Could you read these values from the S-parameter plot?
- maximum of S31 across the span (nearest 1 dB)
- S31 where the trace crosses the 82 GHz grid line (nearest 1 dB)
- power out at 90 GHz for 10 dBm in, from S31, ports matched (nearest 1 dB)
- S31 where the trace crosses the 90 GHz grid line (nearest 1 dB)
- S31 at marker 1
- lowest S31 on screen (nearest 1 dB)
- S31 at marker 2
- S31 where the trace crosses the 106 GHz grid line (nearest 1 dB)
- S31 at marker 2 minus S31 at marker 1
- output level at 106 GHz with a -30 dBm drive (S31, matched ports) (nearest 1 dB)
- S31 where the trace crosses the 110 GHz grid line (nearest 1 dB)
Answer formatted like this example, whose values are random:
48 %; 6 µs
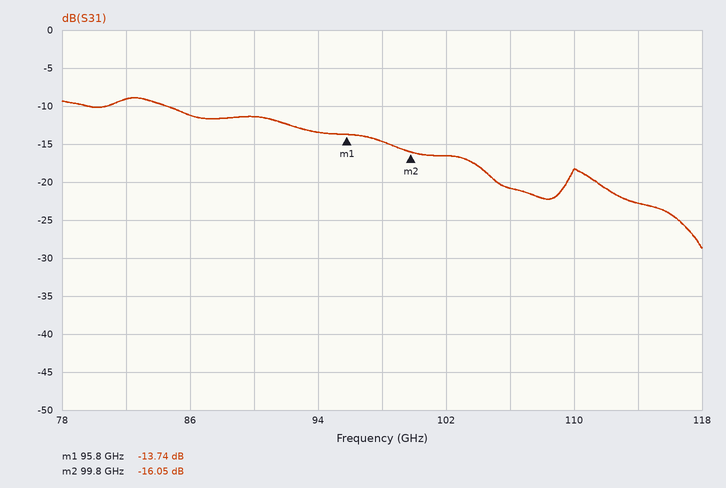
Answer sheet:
-9 dB; -9 dB; -1 dBm; -11 dB; -13.74 dB; -29 dB; -16.05 dB; -21 dB; -2.31 dB; -51 dBm; -18 dB
